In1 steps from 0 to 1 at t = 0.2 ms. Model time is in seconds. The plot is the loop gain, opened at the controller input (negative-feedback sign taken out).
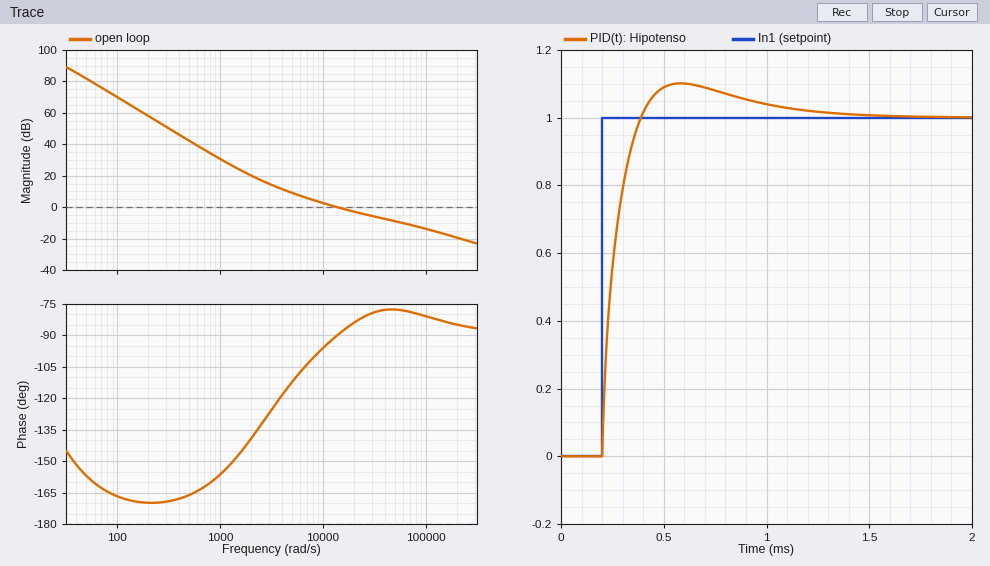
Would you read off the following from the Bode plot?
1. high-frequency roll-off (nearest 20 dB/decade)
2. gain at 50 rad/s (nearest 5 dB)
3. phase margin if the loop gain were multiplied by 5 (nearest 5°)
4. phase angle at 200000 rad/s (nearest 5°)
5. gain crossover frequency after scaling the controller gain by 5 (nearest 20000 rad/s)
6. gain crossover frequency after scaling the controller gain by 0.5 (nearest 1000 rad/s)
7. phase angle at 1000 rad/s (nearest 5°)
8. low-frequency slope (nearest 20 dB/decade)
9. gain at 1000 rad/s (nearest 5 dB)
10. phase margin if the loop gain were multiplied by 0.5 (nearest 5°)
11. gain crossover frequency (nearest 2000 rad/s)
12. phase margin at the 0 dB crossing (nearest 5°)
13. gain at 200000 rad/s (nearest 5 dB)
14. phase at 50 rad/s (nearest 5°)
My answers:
-20 dB/decade
80 dB
100°
-85°
100000 rad/s
7000 rad/s
-155°
-40 dB/decade
30 dB
75°
14000 rad/s
90°
-20 dB
-155°
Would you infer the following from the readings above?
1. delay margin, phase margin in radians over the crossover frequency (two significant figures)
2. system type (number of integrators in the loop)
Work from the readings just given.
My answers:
0.00011 s
2
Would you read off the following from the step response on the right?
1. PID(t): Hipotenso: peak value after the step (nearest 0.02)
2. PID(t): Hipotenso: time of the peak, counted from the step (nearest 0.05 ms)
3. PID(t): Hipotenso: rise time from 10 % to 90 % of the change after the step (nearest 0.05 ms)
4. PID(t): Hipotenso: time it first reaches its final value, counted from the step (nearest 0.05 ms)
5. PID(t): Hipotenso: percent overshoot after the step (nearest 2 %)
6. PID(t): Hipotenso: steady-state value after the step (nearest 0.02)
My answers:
1.10
0.40 ms
0.15 ms
0.20 ms
10 %
1.00
